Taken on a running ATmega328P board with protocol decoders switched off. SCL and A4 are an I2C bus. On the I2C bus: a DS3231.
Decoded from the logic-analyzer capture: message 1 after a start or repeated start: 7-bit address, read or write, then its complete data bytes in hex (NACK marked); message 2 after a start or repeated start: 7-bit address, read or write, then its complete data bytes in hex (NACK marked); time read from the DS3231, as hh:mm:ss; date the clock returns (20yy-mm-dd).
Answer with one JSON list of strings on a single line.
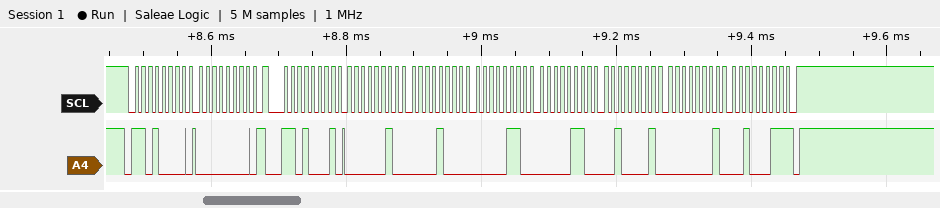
["0x68 write: 00", "0x68 read: 02 08 06 06 21 01 23 NACK", "06:08:02", "2023-01-21"]
